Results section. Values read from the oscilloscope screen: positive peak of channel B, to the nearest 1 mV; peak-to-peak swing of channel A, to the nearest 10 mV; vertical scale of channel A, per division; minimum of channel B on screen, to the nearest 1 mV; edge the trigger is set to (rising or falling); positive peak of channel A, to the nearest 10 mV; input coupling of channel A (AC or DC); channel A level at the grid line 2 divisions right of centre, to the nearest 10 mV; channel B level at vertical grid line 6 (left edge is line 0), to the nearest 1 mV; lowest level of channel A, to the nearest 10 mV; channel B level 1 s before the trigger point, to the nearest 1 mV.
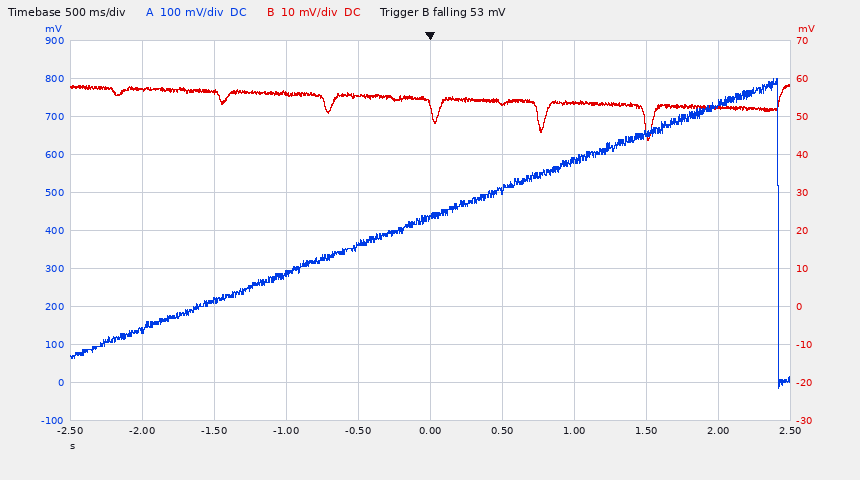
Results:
58 mV
820 mV
100 mV
44 mV
falling
800 mV
DC
580 mV
53 mV
-20 mV
56 mV
